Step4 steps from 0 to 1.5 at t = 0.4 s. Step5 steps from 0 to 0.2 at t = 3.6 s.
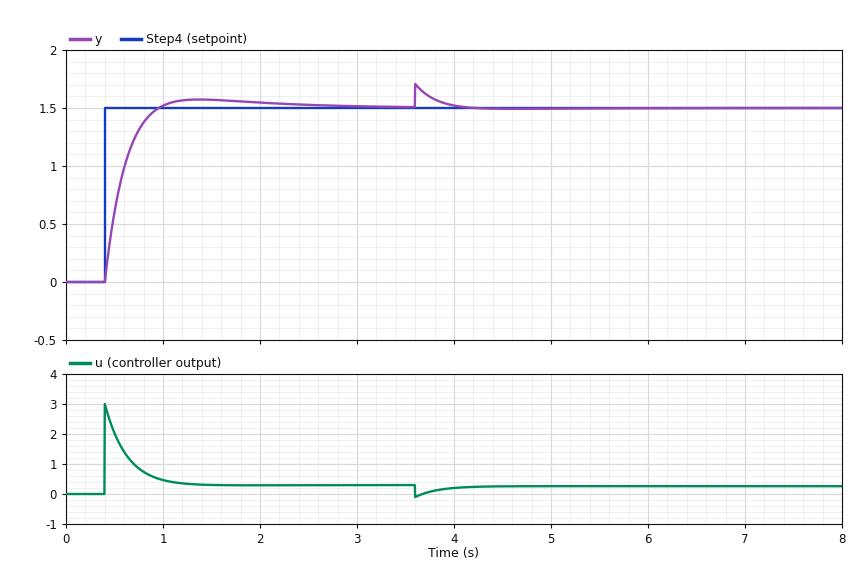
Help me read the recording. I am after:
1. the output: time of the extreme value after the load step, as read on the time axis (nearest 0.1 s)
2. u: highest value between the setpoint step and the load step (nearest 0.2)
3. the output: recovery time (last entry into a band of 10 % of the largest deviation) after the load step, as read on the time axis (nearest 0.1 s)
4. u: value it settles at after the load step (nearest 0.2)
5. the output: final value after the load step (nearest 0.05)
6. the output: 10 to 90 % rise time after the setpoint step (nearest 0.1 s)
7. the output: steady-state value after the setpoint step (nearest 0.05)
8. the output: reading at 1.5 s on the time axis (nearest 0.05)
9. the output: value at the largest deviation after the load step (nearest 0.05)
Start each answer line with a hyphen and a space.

- 3.6 s
- 3.0
- 4.0 s
- 0.2
- 1.50
- 0.4 s
- 1.50
- 1.55
- 1.70
